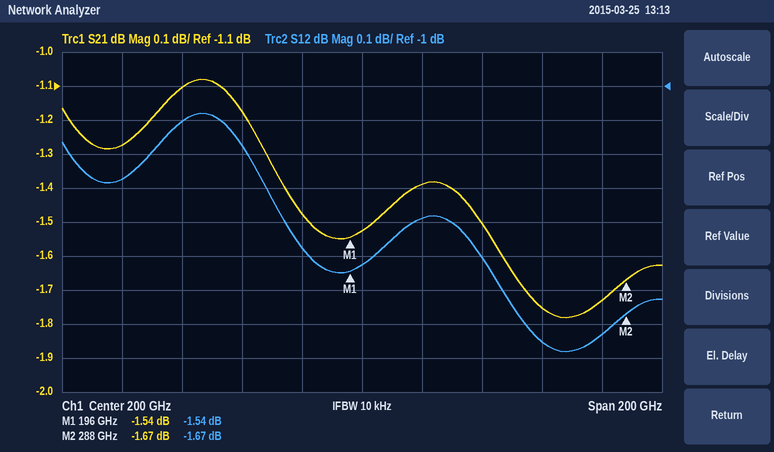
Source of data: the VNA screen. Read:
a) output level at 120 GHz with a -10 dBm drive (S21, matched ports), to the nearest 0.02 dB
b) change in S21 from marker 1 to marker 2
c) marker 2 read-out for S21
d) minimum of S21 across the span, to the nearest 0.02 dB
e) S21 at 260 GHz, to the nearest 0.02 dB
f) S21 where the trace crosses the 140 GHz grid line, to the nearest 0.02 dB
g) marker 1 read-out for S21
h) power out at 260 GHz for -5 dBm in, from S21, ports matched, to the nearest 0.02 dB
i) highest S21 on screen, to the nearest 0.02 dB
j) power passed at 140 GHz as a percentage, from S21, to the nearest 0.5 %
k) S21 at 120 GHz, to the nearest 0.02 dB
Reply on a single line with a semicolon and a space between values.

-11.28 dBm; -0.13 dB; -1.67 dB; -1.78 dB; -1.76 dB; -1.10 dB; -1.54 dB; -6.76 dBm; -1.08 dB; 77.5 %; -1.28 dB
